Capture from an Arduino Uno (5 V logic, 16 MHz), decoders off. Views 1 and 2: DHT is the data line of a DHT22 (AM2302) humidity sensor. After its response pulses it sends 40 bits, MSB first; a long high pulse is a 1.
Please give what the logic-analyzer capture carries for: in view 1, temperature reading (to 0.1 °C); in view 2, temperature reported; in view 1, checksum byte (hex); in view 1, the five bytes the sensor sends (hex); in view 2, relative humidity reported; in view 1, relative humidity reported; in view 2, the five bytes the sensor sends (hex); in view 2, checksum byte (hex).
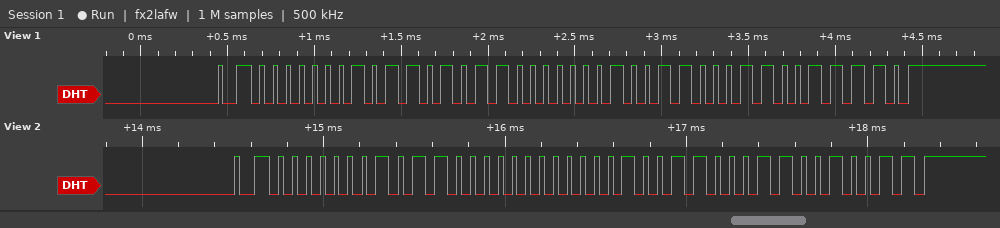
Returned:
30.5 °C
30.5 °C
0x9E
01 6B 01 31 9E
35.2 %
36.3 %
01 60 01 31 93
0x93
